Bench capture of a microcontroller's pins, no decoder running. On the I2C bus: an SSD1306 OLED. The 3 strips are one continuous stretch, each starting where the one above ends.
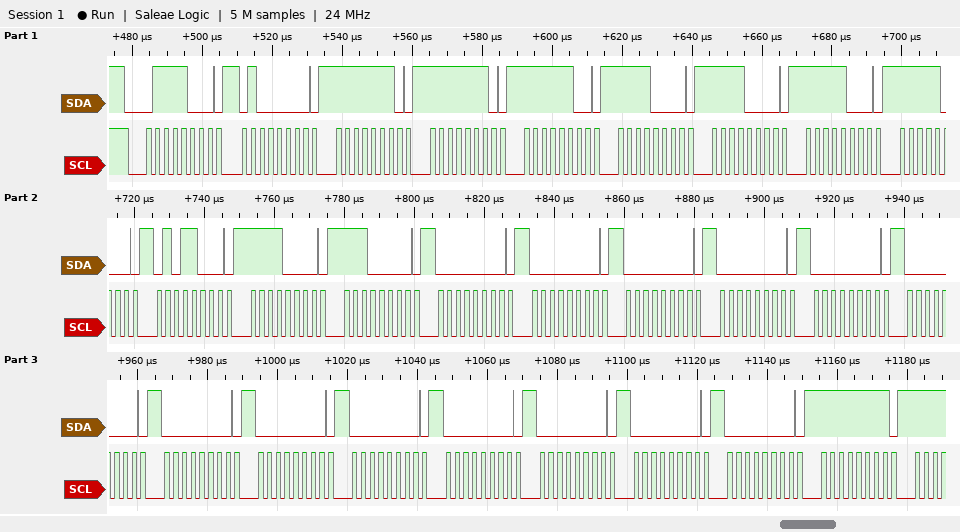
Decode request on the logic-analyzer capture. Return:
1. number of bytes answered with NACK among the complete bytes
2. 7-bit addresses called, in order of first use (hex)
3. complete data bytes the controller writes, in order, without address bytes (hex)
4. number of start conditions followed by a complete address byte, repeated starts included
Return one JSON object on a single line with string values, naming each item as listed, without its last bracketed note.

{"number of bytes answered with NACK among the complete bytes": "0", "7-bit addresses called, in order of first use": "0x3C", "complete data bytes the controller writes, in order, without address bytes": "40 FE FE FC F0 F0 F8 F8 58 F0 E0 00 00 00 00 00 00 00 00 00 00 00 00 00 FF", "number of start conditions followed by a complete address byte, repeated starts included": "1"}
